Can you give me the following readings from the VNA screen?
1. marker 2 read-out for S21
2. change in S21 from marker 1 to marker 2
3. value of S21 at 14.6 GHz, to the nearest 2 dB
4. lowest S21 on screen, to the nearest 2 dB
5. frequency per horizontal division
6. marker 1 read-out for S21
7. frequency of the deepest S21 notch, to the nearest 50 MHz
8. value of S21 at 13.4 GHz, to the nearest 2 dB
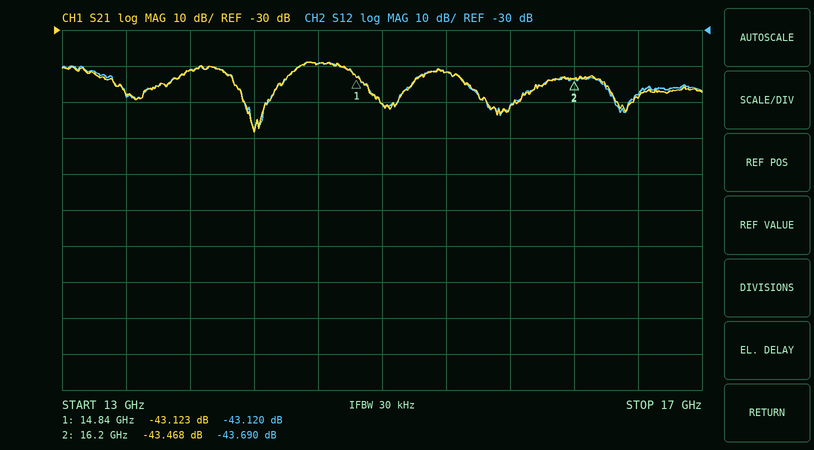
-43.468 dB
-0.345 dB
-40 dB
-58 dB
400 MHz
-43.123 dB
14.20 GHz
-48 dB
